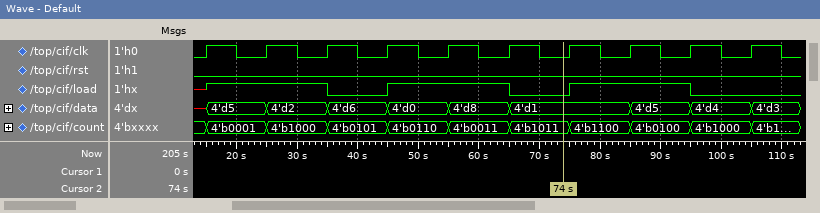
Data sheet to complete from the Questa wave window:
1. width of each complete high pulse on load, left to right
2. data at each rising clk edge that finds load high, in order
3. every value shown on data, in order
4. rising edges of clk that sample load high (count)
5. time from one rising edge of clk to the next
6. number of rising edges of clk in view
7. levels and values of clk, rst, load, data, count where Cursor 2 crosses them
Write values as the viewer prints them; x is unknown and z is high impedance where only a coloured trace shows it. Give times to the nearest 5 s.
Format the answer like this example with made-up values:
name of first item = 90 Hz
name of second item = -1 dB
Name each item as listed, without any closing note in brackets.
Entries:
width of each complete high pulse on load, left to right = 20 s, 20 s
data at each rising clk edge that finds load high, in order = 4'd5, 4'd2, 4'd0, 4'd8, 4'd1, 4'd5
every value shown on data, in order = x, 4'd5, 4'd2, 4'd6, 4'd0, 4'd8, 4'd1, 4'd5, 4'd4, 4'd3
rising edges of clk that sample load high = 6
time from one rising edge of clk to the next = 10 s
number of rising edges of clk in view = 10
levels and values of clk, rst, load, data, count where Cursor 2 crosses them = clk=0, rst=0, load=0, data=4'd1, count=4'b1011
